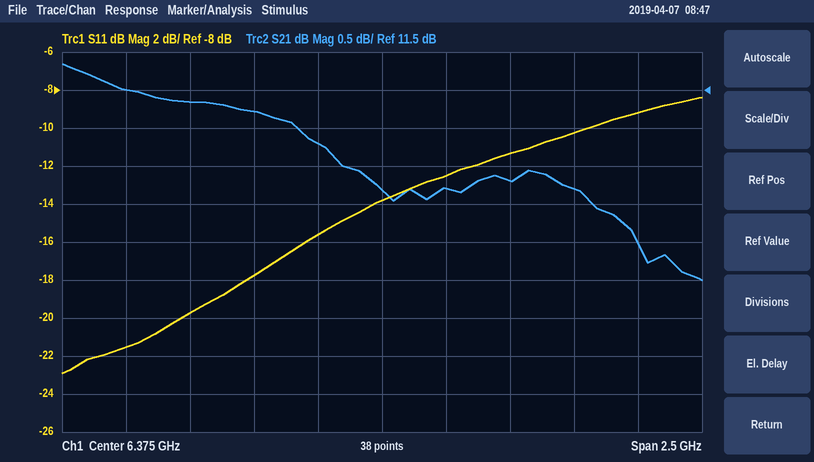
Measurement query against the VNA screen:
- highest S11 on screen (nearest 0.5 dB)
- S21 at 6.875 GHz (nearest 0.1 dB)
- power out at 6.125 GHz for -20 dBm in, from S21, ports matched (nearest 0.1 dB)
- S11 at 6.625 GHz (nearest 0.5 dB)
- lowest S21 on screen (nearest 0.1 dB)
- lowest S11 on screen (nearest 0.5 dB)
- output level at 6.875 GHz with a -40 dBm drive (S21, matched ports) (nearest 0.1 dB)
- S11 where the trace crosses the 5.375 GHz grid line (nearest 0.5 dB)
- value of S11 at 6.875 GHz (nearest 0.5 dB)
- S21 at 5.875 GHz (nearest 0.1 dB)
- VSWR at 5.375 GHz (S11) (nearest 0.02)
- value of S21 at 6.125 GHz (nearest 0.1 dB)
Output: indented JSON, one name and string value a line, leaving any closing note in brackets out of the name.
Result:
{
  "highest S11 on screen": "-8.5 dB",
  "S21 at 6.875 GHz": "10.3 dB",
  "power out at 6.125 GHz for -20 dBm in, from S21, ports matched": "-9.2 dBm",
  "S11 at 6.625 GHz": "-12.5 dB",
  "lowest S21 on screen": "9.0 dB",
  "lowest S11 on screen": "-23.0 dB",
  "output level at 6.875 GHz with a -40 dBm drive (S21, matched ports)": "-29.7 dBm",
  "S11 where the trace crosses the 5.375 GHz grid line": "-21.5 dB",
  "value of S11 at 6.875 GHz": "-11.5 dB",
  "S21 at 5.875 GHz": "11.2 dB",
  "VSWR at 5.375 GHz (S11)": "1.18",
  "value of S21 at 6.125 GHz": "10.8 dB"
}
